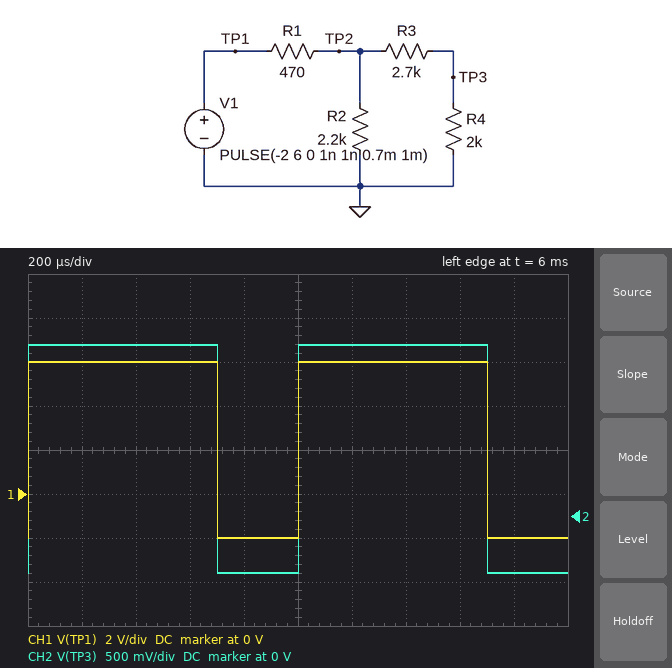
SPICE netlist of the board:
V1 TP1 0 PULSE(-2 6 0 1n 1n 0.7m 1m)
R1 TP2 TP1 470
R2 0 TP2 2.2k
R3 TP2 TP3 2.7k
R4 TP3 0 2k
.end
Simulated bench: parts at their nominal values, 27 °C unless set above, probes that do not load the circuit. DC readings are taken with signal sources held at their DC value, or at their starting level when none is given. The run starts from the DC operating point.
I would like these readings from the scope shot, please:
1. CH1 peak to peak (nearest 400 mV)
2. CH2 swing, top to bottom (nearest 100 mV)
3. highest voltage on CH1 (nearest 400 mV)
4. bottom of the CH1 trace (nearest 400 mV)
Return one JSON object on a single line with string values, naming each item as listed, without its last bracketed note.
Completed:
{"CH1 peak to peak": "8.0 V", "CH2 swing, top to bottom": "2.6 V", "highest voltage on CH1": "6.0 V", "bottom of the CH1 trace": "-2.0 V"}
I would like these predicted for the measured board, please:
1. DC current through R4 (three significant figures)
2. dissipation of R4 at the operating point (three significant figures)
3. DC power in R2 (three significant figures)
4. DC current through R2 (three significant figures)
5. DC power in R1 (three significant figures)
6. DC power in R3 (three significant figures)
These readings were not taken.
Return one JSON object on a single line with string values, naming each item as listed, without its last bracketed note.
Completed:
{"DC current through R4": "324 µA", "dissipation of R4 at the operating point": "210 µW", "DC power in R2": "1.05 mW", "DC current through R2": "692 µA", "DC power in R1": "485 µW", "DC power in R3": "283 µW"}
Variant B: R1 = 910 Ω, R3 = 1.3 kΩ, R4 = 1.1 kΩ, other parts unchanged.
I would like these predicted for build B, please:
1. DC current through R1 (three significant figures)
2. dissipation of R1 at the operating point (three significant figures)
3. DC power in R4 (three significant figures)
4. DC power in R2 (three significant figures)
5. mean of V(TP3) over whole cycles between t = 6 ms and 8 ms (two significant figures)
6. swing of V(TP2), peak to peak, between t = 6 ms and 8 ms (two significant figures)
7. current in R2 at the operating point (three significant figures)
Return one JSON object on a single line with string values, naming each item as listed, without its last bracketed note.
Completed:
{"DC current through R1": "972 µA", "dissipation of R1 at the operating point": "860 µW", "DC power in R4": "238 µW", "DC power in R2": "566 µW", "mean of V(TP3) over whole cycles between t = 6 ms and 8 ms": "920 mV", "swing of V(TP2), peak to peak, between t = 6 ms and 8 ms": "4.5 V", "current in R2 at the operating point": "507 µA"}
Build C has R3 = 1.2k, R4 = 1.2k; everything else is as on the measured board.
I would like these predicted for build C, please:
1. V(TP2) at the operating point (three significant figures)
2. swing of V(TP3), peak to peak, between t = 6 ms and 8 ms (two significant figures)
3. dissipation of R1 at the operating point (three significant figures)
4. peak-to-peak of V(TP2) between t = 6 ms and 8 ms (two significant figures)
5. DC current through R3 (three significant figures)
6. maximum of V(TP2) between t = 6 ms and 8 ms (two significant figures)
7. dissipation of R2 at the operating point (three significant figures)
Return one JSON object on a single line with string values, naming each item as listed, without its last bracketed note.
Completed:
{"V(TP2) at the operating point": "-1.42 V", "swing of V(TP3), peak to peak, between t = 6 ms and 8 ms": "2.8 V", "dissipation of R1 at the operating point": "718 µW", "peak-to-peak of V(TP2) between t = 6 ms and 8 ms": "5.7 V", "DC current through R3": "591 µA", "maximum of V(TP2) between t = 6 ms and 8 ms": "4.3 V", "dissipation of R2 at the operating point": "915 µW"}
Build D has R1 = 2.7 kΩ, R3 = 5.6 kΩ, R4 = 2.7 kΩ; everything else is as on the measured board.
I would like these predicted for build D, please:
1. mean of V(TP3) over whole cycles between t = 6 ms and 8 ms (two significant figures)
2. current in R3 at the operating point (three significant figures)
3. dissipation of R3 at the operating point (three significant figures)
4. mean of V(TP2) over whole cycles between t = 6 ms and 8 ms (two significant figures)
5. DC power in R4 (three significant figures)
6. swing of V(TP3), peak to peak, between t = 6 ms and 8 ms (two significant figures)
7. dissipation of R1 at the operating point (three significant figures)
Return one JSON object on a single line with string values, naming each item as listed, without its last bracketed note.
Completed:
{"mean of V(TP3) over whole cycles between t = 6 ms and 8 ms": "460 mV", "current in R3 at the operating point": "94.4 µA", "dissipation of R3 at the operating point": "49.9 µW", "mean of V(TP2) over whole cycles between t = 6 ms and 8 ms": "1.4 V", "DC power in R4": "24.1 µW", "swing of V(TP3), peak to peak, between t = 6 ms and 8 ms": "1.0 V", "dissipation of R1 at the operating point": "548 µW"}
